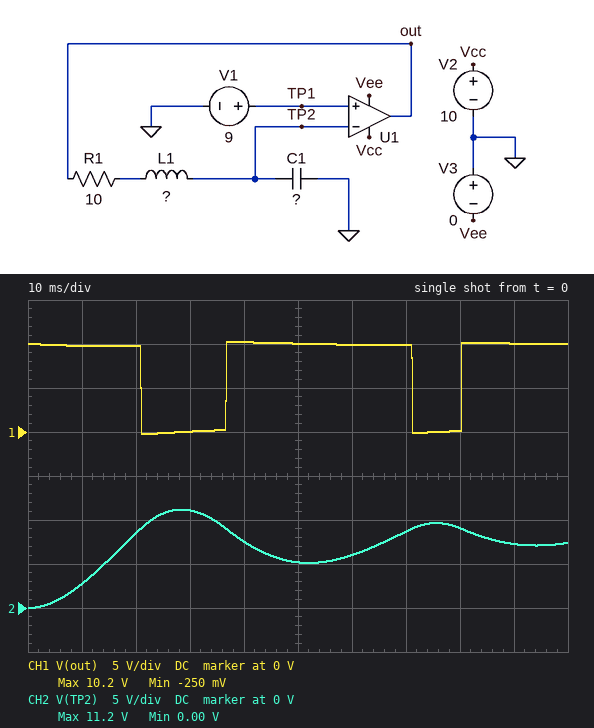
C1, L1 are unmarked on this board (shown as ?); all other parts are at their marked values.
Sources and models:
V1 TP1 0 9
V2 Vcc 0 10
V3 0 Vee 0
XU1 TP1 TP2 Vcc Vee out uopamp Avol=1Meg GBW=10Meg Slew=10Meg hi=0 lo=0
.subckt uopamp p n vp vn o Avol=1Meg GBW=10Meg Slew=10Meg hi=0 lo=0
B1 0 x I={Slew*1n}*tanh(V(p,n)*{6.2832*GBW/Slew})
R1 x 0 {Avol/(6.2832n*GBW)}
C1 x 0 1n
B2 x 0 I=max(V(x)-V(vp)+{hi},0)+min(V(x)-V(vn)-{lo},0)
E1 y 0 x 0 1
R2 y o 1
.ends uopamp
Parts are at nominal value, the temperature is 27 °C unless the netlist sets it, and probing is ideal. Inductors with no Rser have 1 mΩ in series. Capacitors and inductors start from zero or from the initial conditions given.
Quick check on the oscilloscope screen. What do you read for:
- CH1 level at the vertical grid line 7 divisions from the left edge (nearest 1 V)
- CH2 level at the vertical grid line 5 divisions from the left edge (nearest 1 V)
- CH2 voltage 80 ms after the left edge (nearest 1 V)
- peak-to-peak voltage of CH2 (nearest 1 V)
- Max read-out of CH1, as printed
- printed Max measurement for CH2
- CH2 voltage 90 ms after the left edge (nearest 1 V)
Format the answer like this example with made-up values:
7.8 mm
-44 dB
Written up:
10 V
5 V
9 V
11 V
10.2 V
11.2 V
7 V
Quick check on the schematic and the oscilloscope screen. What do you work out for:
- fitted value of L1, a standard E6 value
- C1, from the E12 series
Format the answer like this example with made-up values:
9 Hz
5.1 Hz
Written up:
330 mH
470 µF
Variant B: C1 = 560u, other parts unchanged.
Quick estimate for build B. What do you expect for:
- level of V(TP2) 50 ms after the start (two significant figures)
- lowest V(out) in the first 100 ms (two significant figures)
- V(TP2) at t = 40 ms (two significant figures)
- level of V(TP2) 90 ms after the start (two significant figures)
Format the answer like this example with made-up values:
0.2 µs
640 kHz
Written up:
5.9 V
-290 mV
8.9 V
8.3 V
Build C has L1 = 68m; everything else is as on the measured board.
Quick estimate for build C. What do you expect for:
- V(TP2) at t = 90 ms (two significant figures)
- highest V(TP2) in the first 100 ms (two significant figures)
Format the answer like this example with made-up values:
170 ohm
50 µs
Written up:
9.0 V
9.8 V
